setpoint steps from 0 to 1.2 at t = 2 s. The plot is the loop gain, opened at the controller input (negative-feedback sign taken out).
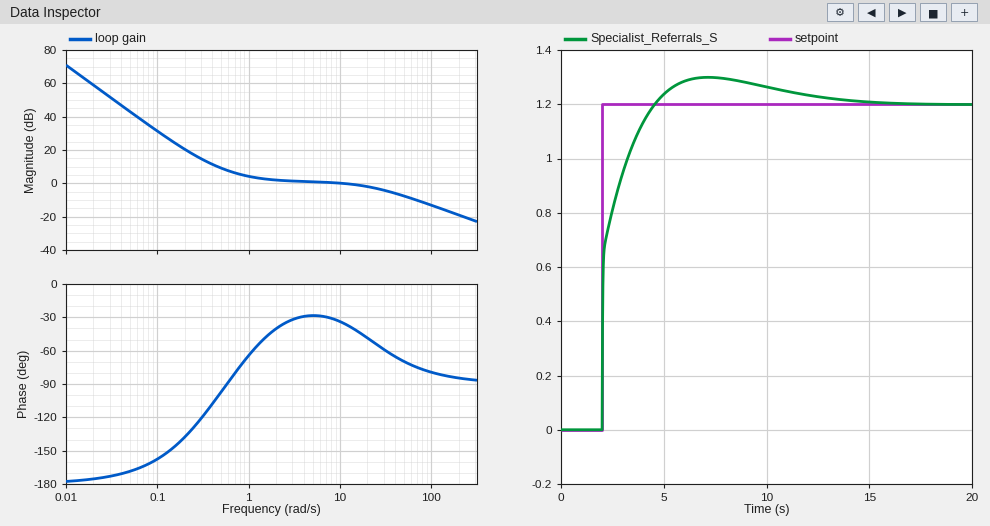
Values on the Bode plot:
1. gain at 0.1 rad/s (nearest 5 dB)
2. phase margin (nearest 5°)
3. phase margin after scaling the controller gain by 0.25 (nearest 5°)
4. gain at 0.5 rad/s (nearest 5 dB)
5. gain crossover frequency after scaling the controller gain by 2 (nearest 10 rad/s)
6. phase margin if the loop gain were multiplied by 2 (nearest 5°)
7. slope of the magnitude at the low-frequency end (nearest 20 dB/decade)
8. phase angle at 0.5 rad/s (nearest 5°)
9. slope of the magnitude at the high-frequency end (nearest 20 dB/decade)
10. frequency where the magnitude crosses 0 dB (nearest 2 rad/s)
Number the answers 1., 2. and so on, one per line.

1. 30 dB
2. 145°
3. 70°
4. 10 dB
5. 40 rad/s
6. 115°
7. -40 dB/decade
8. -95°
9. -20 dB/decade
10. 10 rad/s
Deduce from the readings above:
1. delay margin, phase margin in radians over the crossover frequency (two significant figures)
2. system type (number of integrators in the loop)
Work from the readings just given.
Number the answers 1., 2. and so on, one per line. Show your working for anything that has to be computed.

1. 145 × π / 180 / 10 = 0.25 s
2. 2
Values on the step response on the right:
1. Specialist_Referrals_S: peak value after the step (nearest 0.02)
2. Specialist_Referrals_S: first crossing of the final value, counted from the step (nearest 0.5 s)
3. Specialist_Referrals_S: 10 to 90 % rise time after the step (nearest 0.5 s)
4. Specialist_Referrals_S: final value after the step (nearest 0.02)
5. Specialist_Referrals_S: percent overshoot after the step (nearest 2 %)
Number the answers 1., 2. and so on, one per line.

1. 1.30
2. 2.5 s
3. 1.5 s
4. 1.20
5. 8 %
